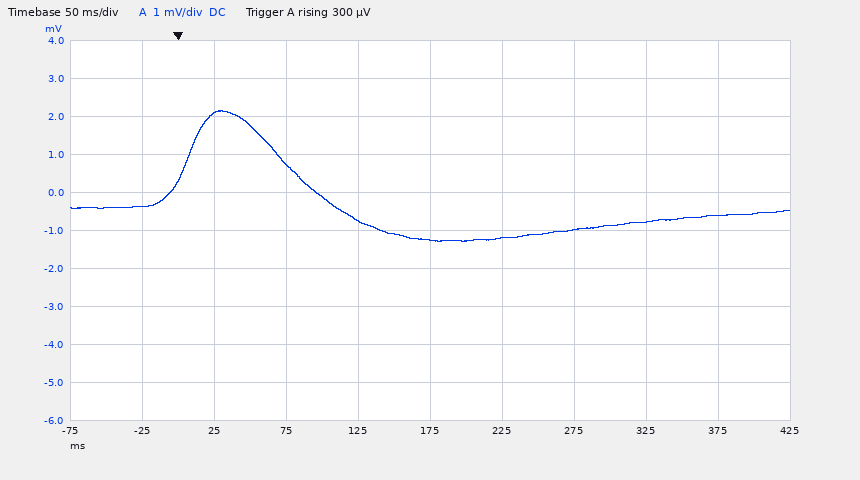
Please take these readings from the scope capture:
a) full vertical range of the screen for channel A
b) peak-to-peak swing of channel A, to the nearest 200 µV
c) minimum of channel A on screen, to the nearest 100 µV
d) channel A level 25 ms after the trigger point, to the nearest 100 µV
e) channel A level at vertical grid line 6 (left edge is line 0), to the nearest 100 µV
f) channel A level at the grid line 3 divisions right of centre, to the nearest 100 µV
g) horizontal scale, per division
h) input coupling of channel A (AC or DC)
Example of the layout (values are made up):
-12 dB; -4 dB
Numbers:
10 mV; 3.4 mV; -1.3 mV; 2.1 mV; -1.2 mV; -800 µV; 50 ms; DC
